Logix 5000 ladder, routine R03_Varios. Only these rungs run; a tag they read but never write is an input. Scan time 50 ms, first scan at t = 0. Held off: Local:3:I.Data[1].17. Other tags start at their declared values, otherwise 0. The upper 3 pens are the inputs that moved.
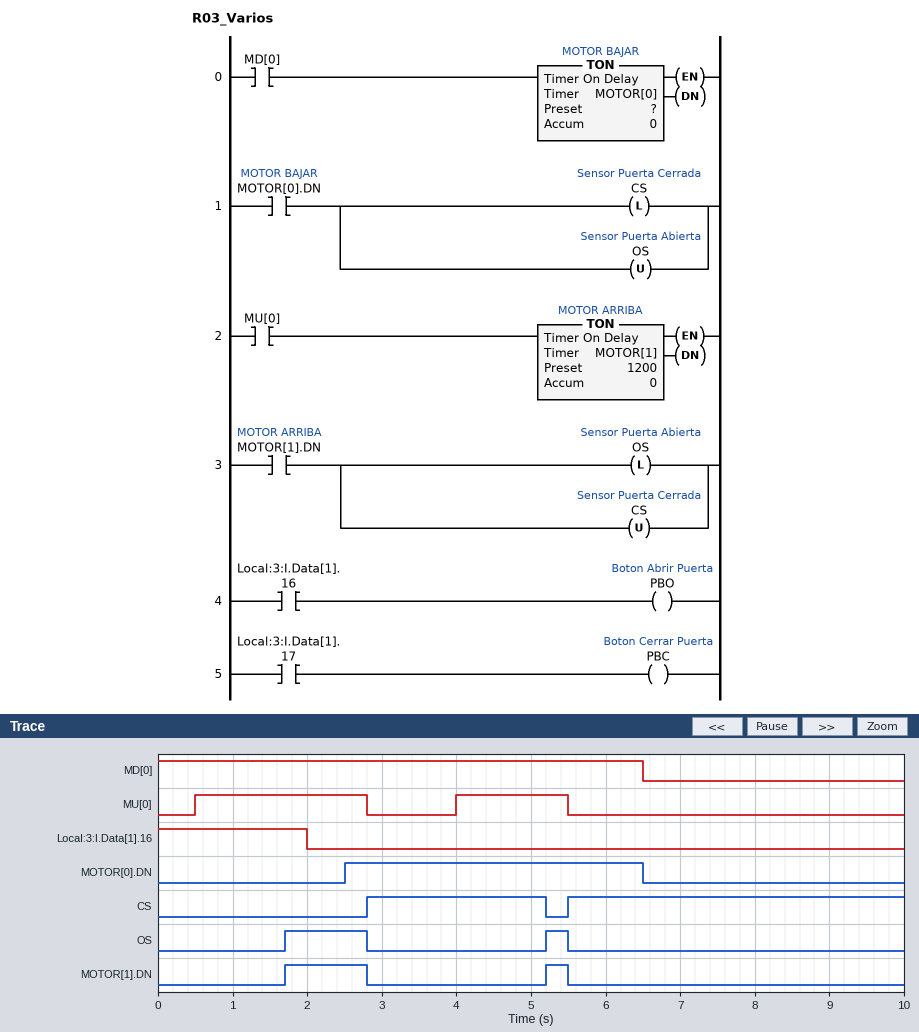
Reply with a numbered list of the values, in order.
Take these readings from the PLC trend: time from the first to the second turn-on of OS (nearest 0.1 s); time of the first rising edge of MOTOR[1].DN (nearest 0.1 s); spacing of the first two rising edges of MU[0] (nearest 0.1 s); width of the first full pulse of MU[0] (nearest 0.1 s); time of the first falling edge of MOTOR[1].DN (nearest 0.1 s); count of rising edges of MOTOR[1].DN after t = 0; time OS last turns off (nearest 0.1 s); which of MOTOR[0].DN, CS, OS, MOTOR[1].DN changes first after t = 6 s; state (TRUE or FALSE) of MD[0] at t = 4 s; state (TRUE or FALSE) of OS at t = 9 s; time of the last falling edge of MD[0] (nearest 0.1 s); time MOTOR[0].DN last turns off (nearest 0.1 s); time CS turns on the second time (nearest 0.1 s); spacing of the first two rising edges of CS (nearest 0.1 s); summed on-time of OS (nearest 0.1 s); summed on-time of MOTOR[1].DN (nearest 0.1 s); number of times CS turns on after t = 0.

1. 3.5 s
2. 1.7 s
3. 3.5 s
4. 2.3 s
5. 2.8 s
6. 2
7. 5.5 s
8. MOTOR[0].DN
9. TRUE
10. FALSE
11. 6.5 s
12. 6.5 s
13. 5.5 s
14. 2.7 s
15. 1.4 s
16. 1.4 s
17. 2
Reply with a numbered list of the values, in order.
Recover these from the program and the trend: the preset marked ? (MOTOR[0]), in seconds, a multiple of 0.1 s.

1. 2.5 s
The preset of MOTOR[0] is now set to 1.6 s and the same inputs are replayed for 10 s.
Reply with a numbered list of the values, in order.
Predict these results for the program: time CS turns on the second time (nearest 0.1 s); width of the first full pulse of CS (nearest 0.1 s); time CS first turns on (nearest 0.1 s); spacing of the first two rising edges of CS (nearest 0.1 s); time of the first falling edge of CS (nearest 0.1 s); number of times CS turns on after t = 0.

1. 2.8 s
2. 0.1 s
3. 1.6 s
4. 1.2 s
5. 1.7 s
6. 3
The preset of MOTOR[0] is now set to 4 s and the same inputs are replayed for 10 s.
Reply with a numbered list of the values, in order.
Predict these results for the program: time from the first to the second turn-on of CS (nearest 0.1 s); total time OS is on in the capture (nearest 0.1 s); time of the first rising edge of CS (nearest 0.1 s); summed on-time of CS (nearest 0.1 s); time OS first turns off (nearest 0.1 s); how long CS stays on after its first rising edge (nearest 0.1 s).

1. 1.5 s
2. 2.6 s
3. 4.0 s
4. 5.7 s
5. 4.0 s
6. 1.2 s
